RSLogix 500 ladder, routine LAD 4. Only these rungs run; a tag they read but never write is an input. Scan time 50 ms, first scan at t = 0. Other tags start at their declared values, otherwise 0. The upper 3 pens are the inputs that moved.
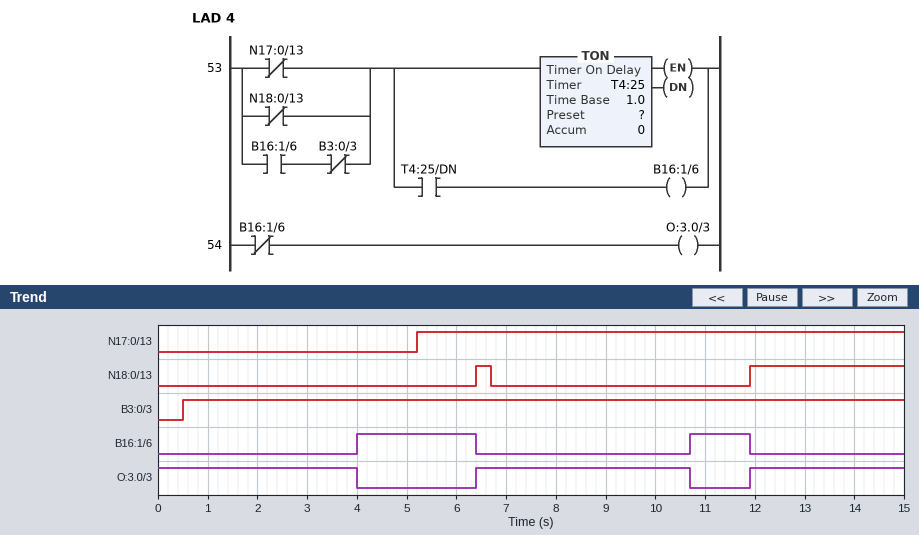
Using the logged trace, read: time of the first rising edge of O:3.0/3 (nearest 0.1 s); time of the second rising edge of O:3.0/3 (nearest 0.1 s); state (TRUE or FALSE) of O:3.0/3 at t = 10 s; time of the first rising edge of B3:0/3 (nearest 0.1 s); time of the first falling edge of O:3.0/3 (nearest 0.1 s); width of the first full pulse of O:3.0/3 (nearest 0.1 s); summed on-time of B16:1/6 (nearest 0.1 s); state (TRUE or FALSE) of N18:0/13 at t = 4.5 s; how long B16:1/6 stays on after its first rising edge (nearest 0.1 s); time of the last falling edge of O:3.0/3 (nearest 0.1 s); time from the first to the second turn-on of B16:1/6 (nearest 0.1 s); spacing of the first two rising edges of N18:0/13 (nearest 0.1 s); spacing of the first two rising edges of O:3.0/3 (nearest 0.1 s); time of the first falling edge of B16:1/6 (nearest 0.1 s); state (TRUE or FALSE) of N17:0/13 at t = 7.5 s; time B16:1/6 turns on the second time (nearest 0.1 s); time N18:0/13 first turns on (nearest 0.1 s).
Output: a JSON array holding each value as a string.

["6.4 s", "11.9 s", "TRUE", "0.5 s", "4.0 s", "4.3 s", "3.6 s", "FALSE", "2.4 s", "10.7 s", "6.7 s", "5.5 s", "5.5 s", "6.4 s", "TRUE", "10.7 s", "6.4 s"]
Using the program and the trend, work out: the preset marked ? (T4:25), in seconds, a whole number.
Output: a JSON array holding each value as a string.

["4 s"]
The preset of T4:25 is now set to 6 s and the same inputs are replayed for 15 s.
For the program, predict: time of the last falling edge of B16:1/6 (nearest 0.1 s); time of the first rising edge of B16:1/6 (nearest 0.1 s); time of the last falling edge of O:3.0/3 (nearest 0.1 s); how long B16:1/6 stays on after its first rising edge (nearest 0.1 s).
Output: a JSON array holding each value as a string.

["6.4 s", "6.0 s", "6.0 s", "0.4 s"]
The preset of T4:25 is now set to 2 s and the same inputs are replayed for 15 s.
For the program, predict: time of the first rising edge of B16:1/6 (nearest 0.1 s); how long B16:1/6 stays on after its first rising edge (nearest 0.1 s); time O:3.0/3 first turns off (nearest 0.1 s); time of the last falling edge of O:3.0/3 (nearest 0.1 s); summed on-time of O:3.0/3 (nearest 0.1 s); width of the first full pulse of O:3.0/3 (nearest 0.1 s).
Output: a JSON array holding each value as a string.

["2.0 s", "4.4 s", "2.0 s", "8.7 s", "7.4 s", "2.3 s"]
